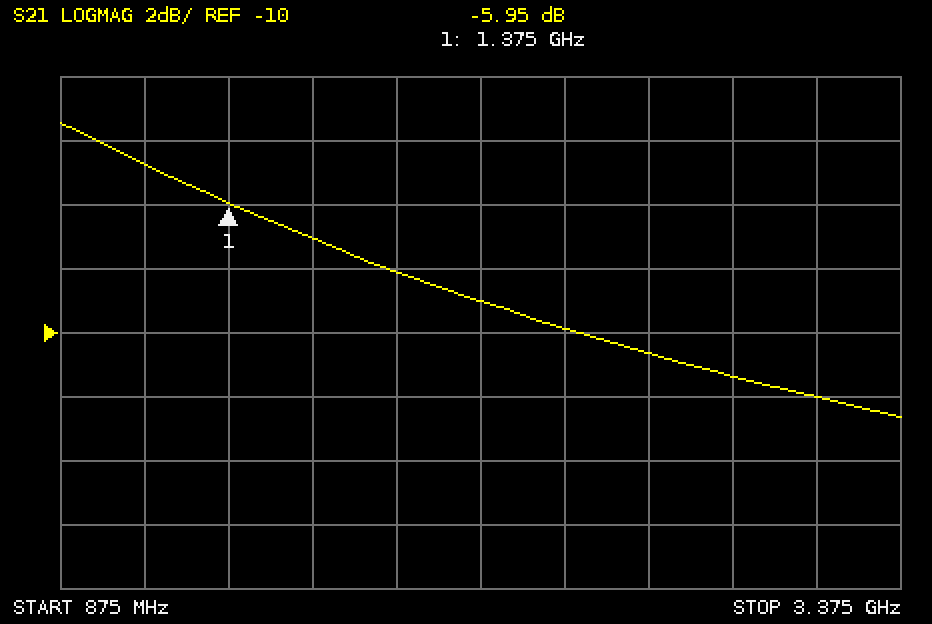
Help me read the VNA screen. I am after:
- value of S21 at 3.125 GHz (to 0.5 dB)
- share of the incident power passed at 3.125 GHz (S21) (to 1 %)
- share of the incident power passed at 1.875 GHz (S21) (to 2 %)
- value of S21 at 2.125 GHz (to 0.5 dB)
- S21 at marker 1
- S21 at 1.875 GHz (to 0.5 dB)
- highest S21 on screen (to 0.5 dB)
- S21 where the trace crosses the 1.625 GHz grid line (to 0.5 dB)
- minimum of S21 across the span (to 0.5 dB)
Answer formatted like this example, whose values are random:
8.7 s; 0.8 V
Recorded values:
-12.0 dB; 6 %; 16 %; -9.0 dB; -5.95 dB; -8.0 dB; -3.5 dB; -7.0 dB; -12.5 dB
